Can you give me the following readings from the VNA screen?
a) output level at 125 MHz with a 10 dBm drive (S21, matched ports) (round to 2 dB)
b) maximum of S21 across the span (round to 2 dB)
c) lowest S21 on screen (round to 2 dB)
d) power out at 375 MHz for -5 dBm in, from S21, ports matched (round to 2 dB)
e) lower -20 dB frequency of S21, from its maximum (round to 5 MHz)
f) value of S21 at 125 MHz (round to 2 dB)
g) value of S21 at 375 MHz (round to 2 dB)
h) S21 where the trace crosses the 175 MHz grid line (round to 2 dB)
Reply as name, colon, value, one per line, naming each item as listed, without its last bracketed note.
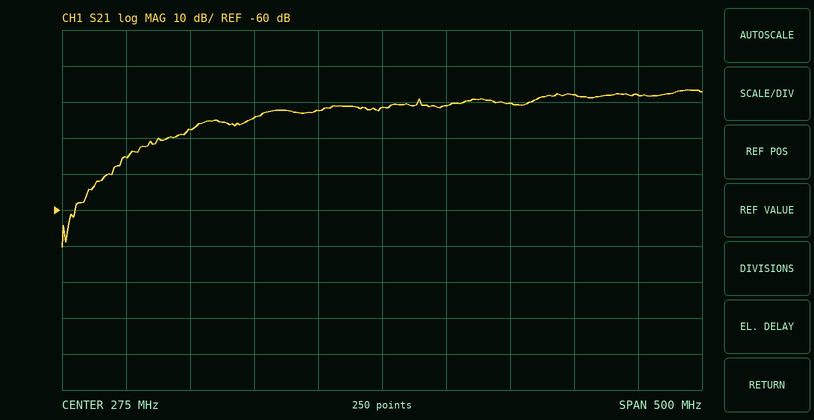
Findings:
output level at 125 MHz with a 10 dBm drive (S21, matched ports): -28 dBm
maximum of S21 across the span: -26 dB
lowest S21 on screen: -70 dB
power out at 375 MHz for -5 dBm in, from S21, ports matched: -36 dBm
lower -20 dB frequency of S21, from its maximum: 70 MHz
value of S21 at 125 MHz: -38 dB
value of S21 at 375 MHz: -30 dB
S21 where the trace crosses the 175 MHz grid line: -34 dB
